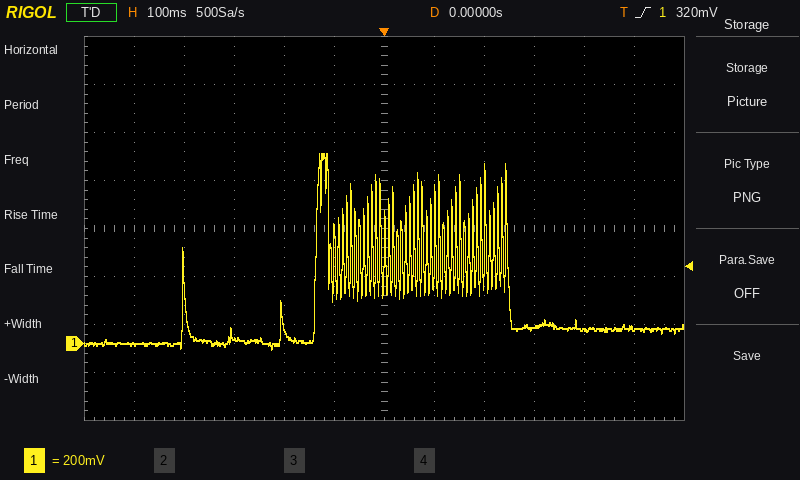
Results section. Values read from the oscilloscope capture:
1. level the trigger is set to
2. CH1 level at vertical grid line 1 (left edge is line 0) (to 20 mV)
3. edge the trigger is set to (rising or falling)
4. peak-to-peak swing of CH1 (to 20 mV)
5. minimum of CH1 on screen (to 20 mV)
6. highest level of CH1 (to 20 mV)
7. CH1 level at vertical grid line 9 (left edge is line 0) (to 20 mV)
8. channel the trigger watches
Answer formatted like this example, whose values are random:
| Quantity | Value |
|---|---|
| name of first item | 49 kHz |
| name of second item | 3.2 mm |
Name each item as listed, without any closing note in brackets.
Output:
| Quantity | Value |
|---|---|
| level the trigger is set to | 320 mV |
| CH1 level at vertical grid line 1 (left edge is line 0) | 0 mV |
| edge the trigger is set to | rising |
| peak-to-peak swing of CH1 | 820 mV |
| minimum of CH1 on screen | -20 mV |
| highest level of CH1 | 800 mV |
| CH1 level at vertical grid line 9 (left edge is line 0) | 60 mV |
| channel the trigger watches | CH1 |
